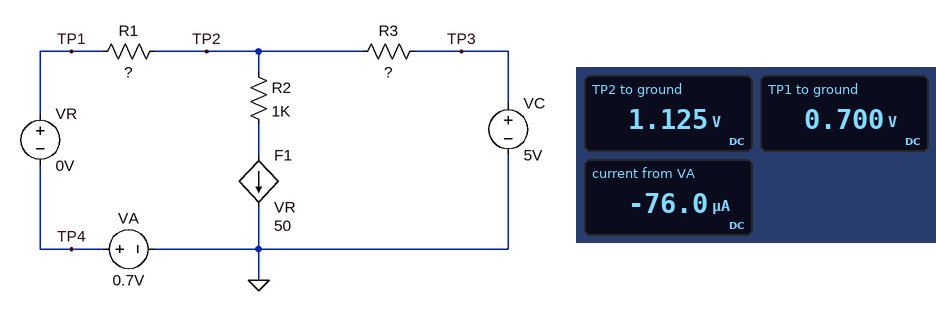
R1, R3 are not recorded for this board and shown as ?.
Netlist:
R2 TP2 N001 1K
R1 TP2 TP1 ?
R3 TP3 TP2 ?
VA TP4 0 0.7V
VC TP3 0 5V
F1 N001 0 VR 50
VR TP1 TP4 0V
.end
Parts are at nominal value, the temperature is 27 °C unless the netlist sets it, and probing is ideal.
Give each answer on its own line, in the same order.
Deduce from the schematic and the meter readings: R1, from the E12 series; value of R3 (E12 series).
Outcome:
5.6 kΩ
1 kΩ
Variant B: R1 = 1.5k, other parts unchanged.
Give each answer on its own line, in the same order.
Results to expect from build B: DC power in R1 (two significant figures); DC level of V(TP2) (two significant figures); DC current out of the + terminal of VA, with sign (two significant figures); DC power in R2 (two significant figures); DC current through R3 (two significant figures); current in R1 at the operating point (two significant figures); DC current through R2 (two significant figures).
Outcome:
10 µW
820 mV
-82 µA
17 mW
4.2 mA
82 µA
4.1 mA
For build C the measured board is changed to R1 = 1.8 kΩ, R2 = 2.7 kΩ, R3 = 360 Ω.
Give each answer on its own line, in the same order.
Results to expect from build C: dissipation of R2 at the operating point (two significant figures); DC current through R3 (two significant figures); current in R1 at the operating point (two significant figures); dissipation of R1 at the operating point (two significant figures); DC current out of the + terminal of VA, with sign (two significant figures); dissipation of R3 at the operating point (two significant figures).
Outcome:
310 mW
11 mA
210 µA
82 µW
-210 µA
43 mW
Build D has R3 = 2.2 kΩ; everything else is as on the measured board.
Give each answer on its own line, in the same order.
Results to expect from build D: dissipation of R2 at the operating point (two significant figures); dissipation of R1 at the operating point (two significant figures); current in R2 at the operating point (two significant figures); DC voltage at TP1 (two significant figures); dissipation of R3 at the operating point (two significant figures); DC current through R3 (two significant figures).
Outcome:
3.3 mW
7.5 µW
1.8 mA
700 mV
7.6 mW
1.9 mA
